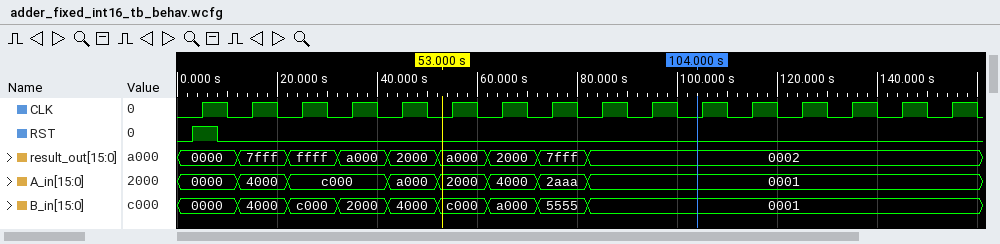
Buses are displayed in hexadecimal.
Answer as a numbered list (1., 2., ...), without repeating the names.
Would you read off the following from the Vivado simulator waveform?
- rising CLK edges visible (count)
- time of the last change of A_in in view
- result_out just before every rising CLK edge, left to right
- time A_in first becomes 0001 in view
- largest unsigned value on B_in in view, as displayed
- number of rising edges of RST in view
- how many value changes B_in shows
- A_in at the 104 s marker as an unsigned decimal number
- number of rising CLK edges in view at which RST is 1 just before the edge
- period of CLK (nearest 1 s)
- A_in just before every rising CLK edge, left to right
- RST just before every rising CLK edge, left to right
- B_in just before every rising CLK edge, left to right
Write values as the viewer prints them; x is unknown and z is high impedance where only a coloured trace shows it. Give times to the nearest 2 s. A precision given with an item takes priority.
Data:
1. 16
2. 82 s
3. 0000, 7fff, ffff, a000, 2000, a000, 2000, 7fff, 0002, 0002, 0002, 0002, 0002, 0002, 0002, 0002
4. 82 s
5. c000
6. 1
7. 8
8. 1
9. 1
10. 10 s
11. 0000, 4000, c000, c000, a000, 2000, 4000, 2aaa, 0001, 0001, 0001, 0001, 0001, 0001, 0001, 0001
12. 1 0 0 0 0 0 0 0 0 0 0 0 0 0 0 0
13. 0000, 4000, c000, 2000, 4000, c000, a000, 5555, 0001, 0001, 0001, 0001, 0001, 0001, 0001, 0001
